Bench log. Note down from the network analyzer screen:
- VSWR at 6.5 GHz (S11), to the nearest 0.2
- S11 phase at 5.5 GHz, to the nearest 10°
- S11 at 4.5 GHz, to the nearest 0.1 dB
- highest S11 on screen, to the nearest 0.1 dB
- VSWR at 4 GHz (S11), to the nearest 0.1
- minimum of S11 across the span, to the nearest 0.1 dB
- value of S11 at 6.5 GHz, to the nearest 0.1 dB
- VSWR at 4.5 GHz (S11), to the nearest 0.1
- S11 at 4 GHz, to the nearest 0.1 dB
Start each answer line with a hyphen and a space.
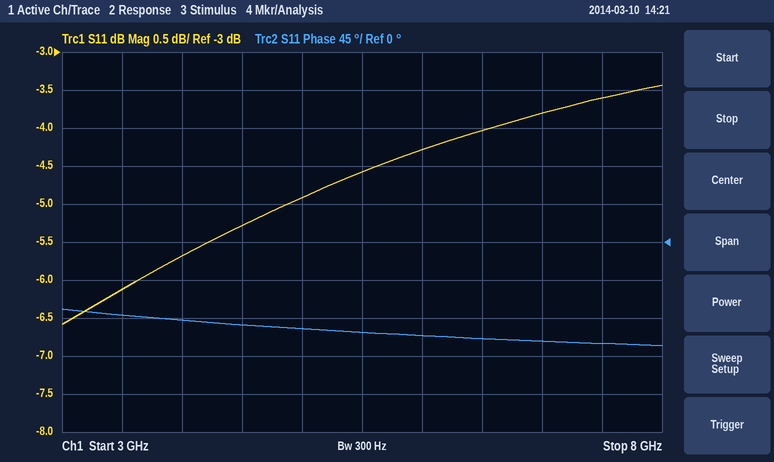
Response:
- 4.4
- -110°
- -5.3 dB
- -3.4 dB
- 3.2
- -6.6 dB
- -4.0 dB
- 3.4
- -5.7 dB
